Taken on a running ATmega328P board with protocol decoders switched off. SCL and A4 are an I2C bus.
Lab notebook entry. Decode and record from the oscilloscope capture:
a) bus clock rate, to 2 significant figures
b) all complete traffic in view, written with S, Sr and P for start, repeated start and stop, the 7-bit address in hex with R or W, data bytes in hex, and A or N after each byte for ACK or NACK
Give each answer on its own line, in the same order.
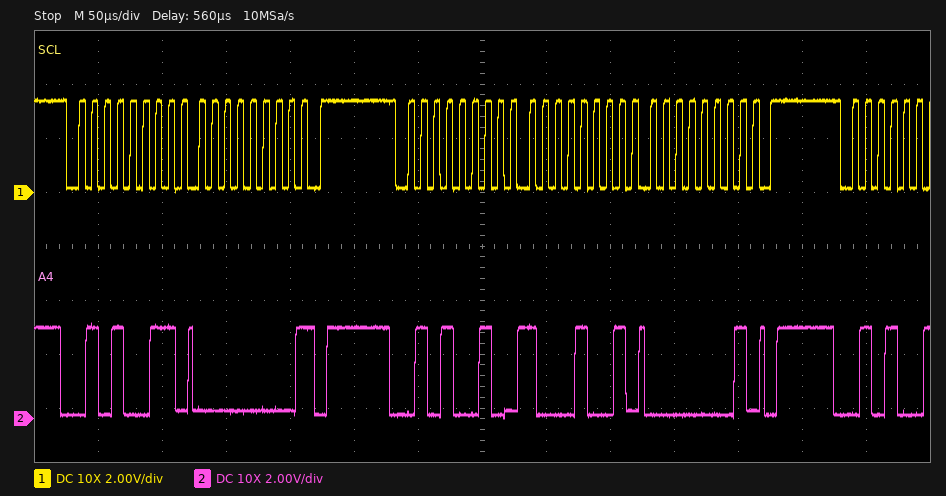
100 kHz
S 29R A 00 N P S 29W A 89 A 01 A P
